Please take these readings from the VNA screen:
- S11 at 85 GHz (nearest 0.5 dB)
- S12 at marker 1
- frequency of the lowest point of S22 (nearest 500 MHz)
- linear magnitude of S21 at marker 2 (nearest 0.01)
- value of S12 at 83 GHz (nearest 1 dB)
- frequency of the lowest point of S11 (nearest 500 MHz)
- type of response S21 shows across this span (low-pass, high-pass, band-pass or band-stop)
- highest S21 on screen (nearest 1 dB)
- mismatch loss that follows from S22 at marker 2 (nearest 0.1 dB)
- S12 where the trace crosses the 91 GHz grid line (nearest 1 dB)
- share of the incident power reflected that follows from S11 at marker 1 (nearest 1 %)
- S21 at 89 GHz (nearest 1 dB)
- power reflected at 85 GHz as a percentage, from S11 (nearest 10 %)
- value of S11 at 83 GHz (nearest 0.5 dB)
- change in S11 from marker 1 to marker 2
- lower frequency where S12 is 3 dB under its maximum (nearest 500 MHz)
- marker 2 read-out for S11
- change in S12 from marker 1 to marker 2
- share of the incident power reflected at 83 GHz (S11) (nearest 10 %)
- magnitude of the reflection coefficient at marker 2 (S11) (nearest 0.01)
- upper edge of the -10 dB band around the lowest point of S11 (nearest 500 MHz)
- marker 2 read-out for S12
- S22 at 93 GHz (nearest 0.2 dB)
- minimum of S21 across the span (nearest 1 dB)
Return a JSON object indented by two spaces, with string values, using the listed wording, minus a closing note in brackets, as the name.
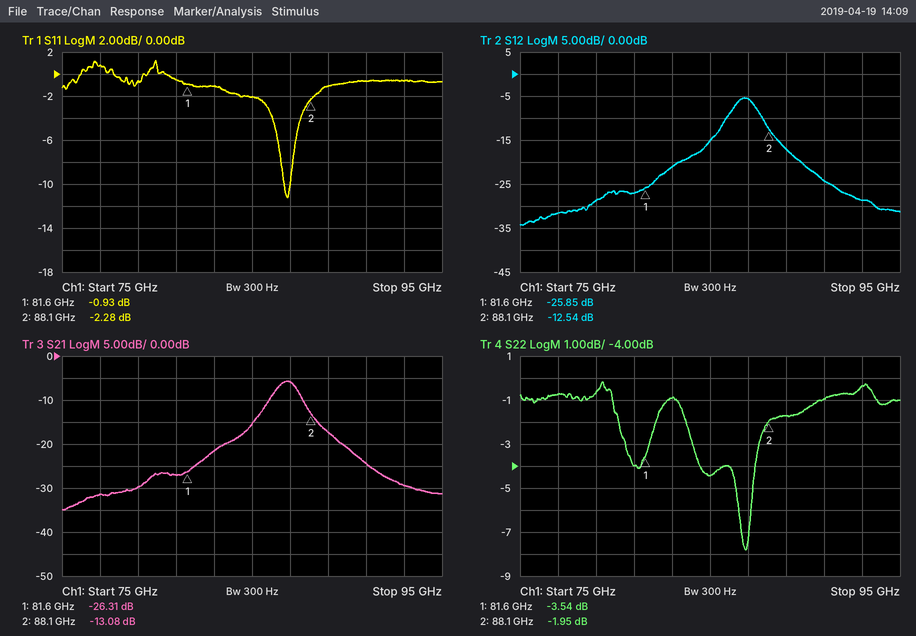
{
  "S11 at 85 GHz": "-2.0 dB",
  "S12 at marker 1": "-25.85 dB",
  "frequency of the lowest point of S22": "87.0 GHz",
  "linear magnitude of S21 at marker 2": "0.22",
  "value of S12 at 83 GHz": "-21 dB",
  "frequency of the lowest point of S11": "87.0 GHz",
  "type of response S21 shows across this span": "band-pass",
  "highest S21 on screen": "-6 dB",
  "mismatch loss that follows from S22 at marker 2": "4.4 dB",
  "S12 where the trace crosses the 91 GHz grid line": "-24 dB",
  "share of the incident power reflected that follows from S11 at marker 1": "81 %",
  "S21 at 89 GHz": "-17 dB",
  "power reflected at 85 GHz as a percentage, from S11": "60 %",
  "value of S11 at 83 GHz": "-1.0 dB",
  "change in S11 from marker 1 to marker 2": "-1.35 dB",
  "lower frequency where S12 is 3 dB under its maximum": "86.0 GHz",
  "marker 2 read-out for S11": "-2.28 dB",
  "change in S12 from marker 1 to marker 2": "13.31 dB",
  "share of the incident power reflected at 83 GHz (S11)": "80 %",
  "magnitude of the reflection coefficient at marker 2 (S11)": "0.77",
  "upper edge of the -10 dB band around the lowest point of S11": "87.0 GHz",
  "marker 2 read-out for S12": "-12.54 dB",
  "S22 at 93 GHz": "-0.4 dB",
  "minimum of S21 across the span": "-35 dB"
}
